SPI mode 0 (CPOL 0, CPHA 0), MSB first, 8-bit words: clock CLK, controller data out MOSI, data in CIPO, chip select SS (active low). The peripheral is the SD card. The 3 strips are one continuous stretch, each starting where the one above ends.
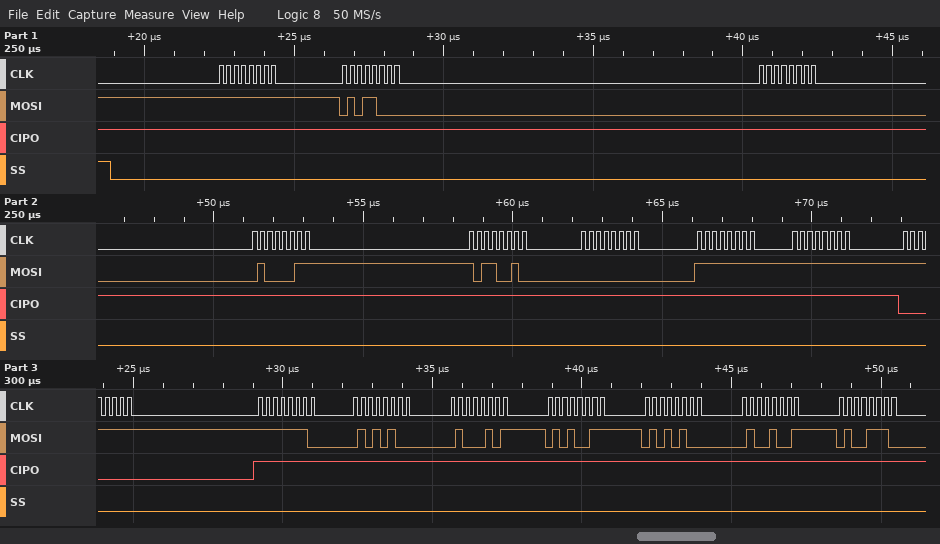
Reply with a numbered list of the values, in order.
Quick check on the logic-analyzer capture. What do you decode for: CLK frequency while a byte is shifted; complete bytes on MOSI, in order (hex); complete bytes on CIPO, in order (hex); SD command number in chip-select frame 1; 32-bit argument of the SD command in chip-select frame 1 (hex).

1. 4 MHz
2. FF 58 00 43 B2 00 FF FF FF FE 54 45 53 54 49 4E
3. FF FF FF FF FF FF FF FF 00 FF FF FF FF FF FF FF
4. CMD24
5. 0x0043B200
